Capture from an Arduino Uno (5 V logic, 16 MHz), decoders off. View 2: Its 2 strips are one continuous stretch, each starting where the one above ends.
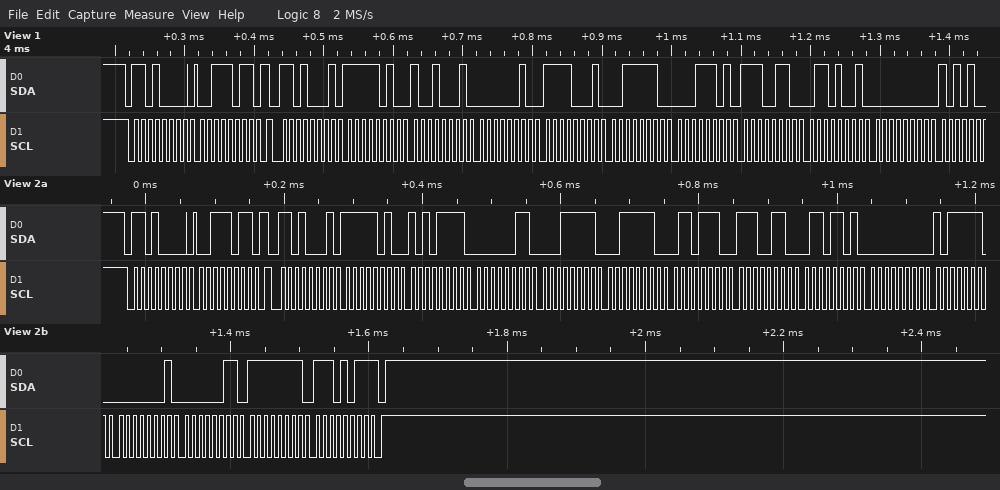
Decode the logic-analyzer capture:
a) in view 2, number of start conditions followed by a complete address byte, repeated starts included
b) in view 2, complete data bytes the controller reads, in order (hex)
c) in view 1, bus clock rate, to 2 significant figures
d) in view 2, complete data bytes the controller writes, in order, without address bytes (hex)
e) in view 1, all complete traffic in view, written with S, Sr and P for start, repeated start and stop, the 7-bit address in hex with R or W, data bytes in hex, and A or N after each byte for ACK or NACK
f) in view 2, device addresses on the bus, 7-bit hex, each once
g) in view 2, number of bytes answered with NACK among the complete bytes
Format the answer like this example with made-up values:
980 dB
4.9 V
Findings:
2
FA AF 03 1F 3E 6E E6 6D 00 BE 01 03 FF EB
100 kHz
3B
S 68W A 3B A Sr 68R A FA A 91 A 02 A F1 A 3E A 1D A E6 A 69 A 00 A
0x68
1
